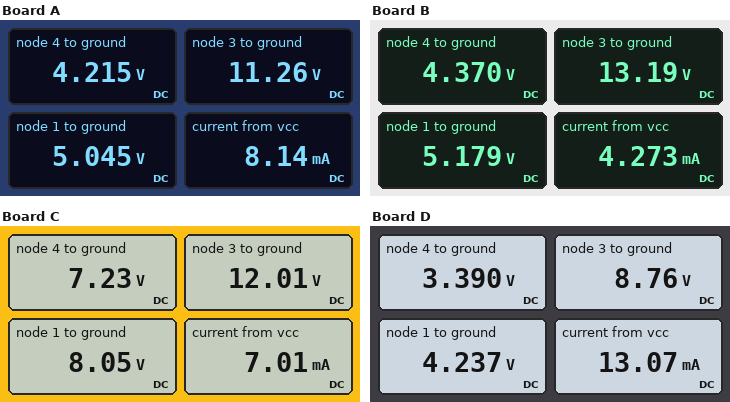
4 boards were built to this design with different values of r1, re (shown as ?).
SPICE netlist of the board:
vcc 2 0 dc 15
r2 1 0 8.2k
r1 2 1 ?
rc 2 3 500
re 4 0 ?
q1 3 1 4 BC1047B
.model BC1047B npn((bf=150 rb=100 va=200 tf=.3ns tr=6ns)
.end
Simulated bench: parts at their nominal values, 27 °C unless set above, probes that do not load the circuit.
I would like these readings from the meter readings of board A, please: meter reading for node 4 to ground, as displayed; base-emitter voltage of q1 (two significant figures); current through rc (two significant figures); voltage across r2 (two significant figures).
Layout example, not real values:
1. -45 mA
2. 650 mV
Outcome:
1. 4.215 V
2. 830 mV
3. 7.5 mA
4. 5.0 V
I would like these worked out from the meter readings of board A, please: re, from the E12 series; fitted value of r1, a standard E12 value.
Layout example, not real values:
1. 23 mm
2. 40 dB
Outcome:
1. 560 Ω
2. 15 kΩ
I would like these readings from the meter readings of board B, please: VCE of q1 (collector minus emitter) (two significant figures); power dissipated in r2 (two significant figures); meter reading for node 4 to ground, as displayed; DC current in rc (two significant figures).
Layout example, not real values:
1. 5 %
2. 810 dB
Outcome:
1. 8.8 V
2. 3.3 mW
3. 4.370 V
4. 3.6 mA
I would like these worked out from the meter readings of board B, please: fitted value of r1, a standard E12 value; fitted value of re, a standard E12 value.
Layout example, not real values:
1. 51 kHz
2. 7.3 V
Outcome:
1. 15 kΩ
2. 1.2 kΩ
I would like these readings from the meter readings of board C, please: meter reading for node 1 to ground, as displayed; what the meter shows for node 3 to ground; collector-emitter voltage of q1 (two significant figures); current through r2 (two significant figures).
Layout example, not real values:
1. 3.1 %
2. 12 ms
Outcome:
1. 8.05 V
2. 12.01 V
3. 4.8 V
4. 980 µA
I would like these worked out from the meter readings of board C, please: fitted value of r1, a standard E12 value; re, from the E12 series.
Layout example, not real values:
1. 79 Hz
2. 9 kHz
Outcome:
1. 6.8 kΩ
2. 1.2 kΩ
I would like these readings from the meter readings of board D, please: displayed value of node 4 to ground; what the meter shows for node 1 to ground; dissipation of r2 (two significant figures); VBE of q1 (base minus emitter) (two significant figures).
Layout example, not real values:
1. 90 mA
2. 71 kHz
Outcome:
1. 3.390 V
2. 4.237 V
3. 2.2 mW
4. 850 mV
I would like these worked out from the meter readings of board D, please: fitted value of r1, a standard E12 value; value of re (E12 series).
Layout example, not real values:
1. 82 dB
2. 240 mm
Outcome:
1. 18 kΩ
2. 270 Ω
